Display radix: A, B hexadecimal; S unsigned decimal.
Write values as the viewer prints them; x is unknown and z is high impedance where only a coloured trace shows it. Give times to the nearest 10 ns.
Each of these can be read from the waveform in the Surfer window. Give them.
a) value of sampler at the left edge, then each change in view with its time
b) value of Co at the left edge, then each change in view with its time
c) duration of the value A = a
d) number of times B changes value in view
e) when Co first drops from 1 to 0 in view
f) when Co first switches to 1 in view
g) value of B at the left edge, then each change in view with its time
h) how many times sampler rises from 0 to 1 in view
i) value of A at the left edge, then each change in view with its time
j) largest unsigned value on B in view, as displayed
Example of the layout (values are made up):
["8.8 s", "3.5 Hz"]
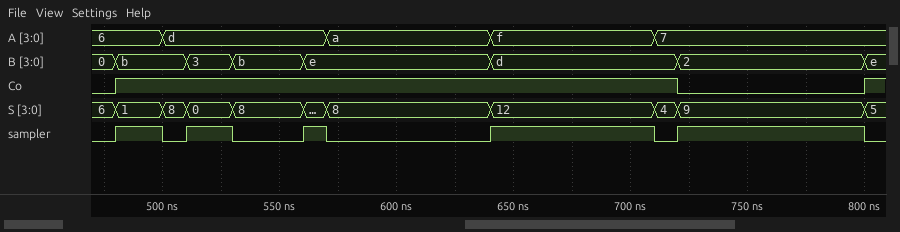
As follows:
["0, 1 at 480 ns, 0 at 500 ns, 1 at 510 ns, 0 at 530 ns, 1 at 560 ns, 0 at 570 ns, 1 at 640 ns, 0 at 710 ns, 1 at 720 ns, 0 at 800 ns", "0, 1 at 480 ns, 0 at 720 ns, 1 at 800 ns", "70 ns", "7", "720 ns", "480 ns", "0, b at 480 ns, 3 at 510 ns, b at 530 ns, e at 560 ns, d at 640 ns, 2 at 720 ns, e at 800 ns", "5", "6, d at 500 ns, a at 570 ns, f at 640 ns, 7 at 710 ns", "e"]
